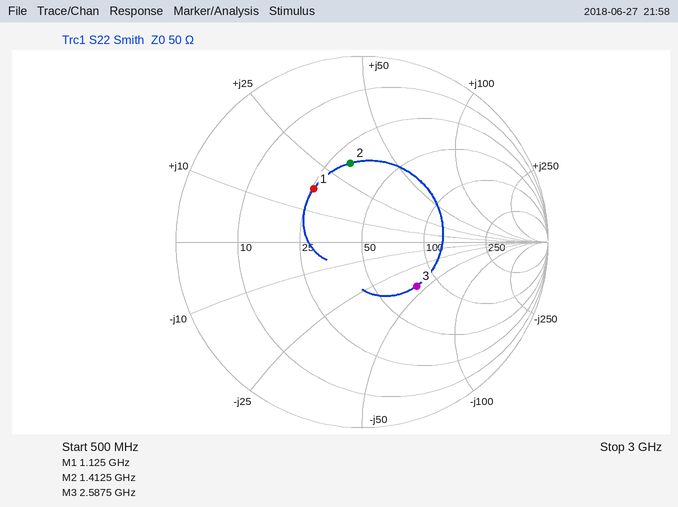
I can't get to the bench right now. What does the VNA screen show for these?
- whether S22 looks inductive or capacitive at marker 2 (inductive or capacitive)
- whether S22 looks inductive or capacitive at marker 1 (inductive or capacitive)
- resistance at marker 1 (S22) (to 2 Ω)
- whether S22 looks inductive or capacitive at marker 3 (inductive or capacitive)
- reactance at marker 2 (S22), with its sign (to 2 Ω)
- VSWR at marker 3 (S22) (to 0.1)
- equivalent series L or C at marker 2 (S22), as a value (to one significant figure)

inductive
inductive
26 Ω
capacitive
+32 Ω
2.2
4 nH
